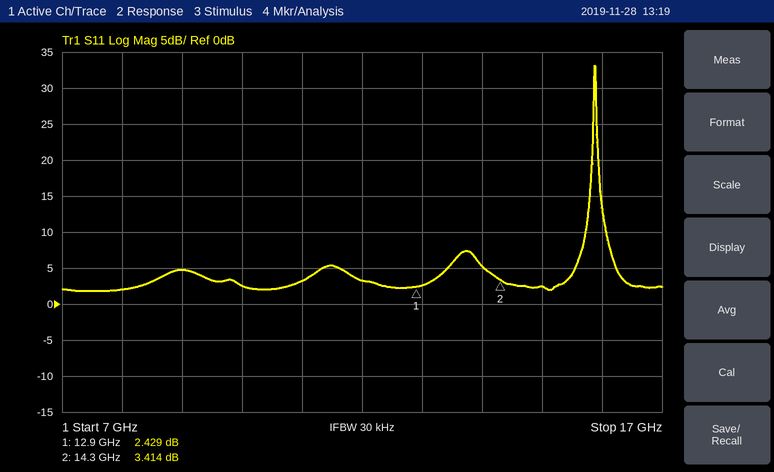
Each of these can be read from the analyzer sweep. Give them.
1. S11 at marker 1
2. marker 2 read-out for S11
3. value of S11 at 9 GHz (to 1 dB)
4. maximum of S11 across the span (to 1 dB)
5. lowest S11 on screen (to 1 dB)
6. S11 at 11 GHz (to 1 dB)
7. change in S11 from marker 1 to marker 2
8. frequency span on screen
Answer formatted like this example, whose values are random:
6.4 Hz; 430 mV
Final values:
2.429 dB; 3.414 dB; 5 dB; 33 dB; 2 dB; 3 dB; 0.985 dB; 10 GHz
